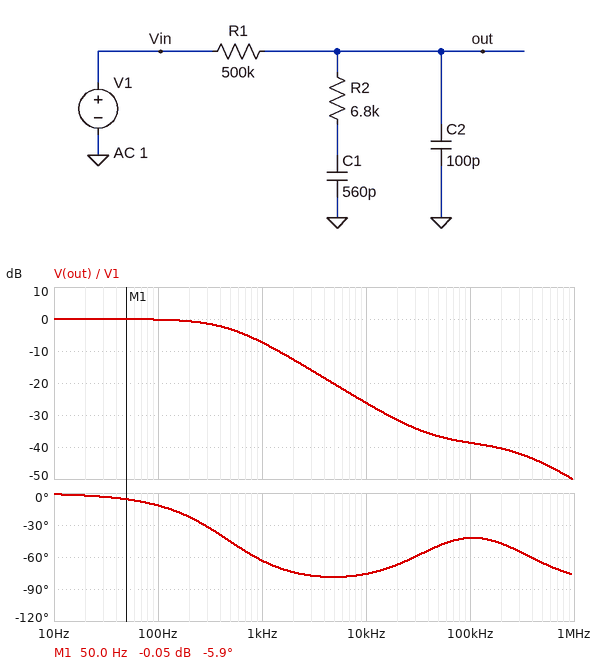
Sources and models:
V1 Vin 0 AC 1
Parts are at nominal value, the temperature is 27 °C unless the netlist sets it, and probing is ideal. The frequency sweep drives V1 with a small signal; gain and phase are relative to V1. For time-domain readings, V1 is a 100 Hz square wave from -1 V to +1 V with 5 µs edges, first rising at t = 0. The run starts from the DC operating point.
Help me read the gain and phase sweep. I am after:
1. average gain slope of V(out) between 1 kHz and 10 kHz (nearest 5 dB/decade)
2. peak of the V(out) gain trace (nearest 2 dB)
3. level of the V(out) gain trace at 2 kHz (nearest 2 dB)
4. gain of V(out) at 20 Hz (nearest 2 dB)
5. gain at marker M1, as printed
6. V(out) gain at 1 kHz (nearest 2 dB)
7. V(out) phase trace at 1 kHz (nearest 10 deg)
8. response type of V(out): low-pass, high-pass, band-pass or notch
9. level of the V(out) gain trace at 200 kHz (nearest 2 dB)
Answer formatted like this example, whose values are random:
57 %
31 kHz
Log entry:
-20 dB/decade
0 dB
-12 dB
0 dB
-0.05 dB
-8 dB
-60 deg
low-pass
-40 dB
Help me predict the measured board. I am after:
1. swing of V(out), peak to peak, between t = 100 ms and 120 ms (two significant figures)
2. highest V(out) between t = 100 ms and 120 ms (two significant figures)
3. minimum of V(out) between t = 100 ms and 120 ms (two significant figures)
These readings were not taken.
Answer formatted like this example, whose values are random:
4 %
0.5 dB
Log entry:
2.0 V
1.0 V
-1.0 V
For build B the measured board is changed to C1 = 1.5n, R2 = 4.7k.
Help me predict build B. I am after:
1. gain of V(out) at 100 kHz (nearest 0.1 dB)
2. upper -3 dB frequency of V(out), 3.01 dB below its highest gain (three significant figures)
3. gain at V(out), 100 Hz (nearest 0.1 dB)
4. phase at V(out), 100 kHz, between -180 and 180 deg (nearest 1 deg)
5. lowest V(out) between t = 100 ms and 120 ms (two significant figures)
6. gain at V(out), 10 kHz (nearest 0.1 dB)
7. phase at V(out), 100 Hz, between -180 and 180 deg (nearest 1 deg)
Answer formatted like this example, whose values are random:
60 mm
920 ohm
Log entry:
-41.3 dB
197 Hz
-1.0 dB
-28 deg
-1.0 V
-33.3 dB
-27 deg
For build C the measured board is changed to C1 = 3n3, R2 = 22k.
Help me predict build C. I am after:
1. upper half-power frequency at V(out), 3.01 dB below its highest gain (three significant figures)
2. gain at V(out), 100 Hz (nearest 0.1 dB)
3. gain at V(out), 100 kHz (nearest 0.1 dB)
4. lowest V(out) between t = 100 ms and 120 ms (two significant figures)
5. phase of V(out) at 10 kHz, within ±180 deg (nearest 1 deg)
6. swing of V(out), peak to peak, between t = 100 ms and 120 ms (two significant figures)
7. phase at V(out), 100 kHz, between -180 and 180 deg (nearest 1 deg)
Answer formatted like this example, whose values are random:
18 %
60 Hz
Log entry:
90.0 Hz
-3.5 dB
-32.0 dB
-890 mV
-19 deg
1.8 V
-53 deg
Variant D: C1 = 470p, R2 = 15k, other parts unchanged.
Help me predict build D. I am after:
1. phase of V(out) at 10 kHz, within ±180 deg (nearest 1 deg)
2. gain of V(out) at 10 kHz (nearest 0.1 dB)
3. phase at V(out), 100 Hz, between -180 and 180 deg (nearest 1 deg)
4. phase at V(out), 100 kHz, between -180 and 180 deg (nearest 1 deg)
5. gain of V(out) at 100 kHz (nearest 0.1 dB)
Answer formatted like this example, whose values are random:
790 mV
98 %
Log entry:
-67 deg
-24.5 dB
-10 deg
-50 deg
-34.1 dB
